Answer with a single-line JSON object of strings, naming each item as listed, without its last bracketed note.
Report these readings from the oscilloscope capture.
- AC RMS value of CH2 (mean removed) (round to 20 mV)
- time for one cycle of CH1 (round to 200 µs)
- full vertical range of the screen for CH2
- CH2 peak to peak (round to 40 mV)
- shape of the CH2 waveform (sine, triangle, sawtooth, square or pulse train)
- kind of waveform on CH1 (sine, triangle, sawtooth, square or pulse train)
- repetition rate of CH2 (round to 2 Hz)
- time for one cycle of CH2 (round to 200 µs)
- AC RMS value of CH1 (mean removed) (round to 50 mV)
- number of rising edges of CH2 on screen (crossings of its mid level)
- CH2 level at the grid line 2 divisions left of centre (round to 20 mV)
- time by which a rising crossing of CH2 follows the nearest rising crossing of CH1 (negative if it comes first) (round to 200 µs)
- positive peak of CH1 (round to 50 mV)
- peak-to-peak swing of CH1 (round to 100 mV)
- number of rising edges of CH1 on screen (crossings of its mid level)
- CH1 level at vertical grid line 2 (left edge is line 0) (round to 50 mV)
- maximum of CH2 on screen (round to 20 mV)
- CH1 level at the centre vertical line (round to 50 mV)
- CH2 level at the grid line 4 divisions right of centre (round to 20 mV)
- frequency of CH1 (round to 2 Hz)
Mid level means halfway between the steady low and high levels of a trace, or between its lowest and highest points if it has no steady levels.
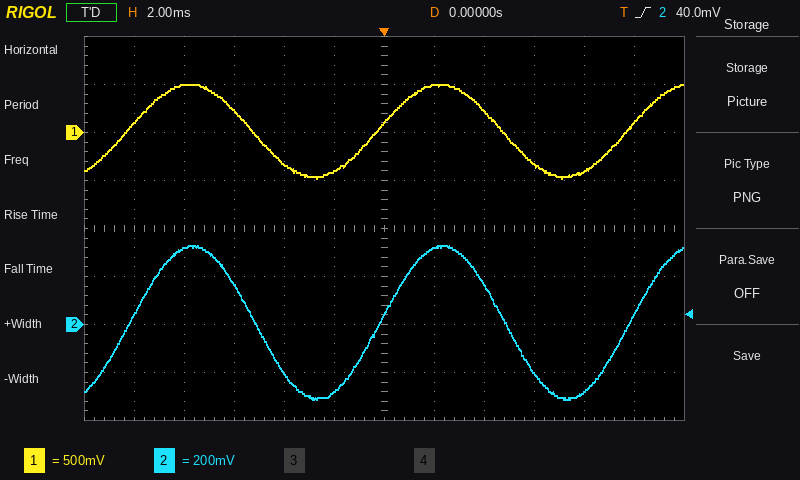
{"AC RMS value of CH2 (mean removed)": "220 mV", "time for one cycle of CH1": "10.0 ms", "full vertical range of the screen for CH2": "1.6 V", "CH2 peak to peak": "640 mV", "shape of the CH2 waveform": "sine", "kind of waveform on CH1": "sine", "repetition rate of CH2": "100 Hz", "time for one cycle of CH2": "10.0 ms", "AC RMS value of CH1 (mean removed)": "350 mV", "number of rising edges of CH2 on screen": "3", "CH2 level at the grid line 2 divisions left of centre": "-200 mV", "time by which a rising crossing of CH2 follows the nearest rising crossing of CH1 (negative if it comes first)": "+200 µs", "positive peak of CH1": "500 mV", "peak-to-peak swing of CH1": "1.00 V", "number of rising edges of CH1 on screen": "3", "CH1 level at vertical grid line 2 (left edge is line 0)": "500 mV", "maximum of CH2 on screen": "320 mV", "CH1 level at the centre vertical line": "100 mV", "CH2 level at the grid line 4 divisions right of centre": "-280 mV", "frequency of CH1": "100 Hz"}
